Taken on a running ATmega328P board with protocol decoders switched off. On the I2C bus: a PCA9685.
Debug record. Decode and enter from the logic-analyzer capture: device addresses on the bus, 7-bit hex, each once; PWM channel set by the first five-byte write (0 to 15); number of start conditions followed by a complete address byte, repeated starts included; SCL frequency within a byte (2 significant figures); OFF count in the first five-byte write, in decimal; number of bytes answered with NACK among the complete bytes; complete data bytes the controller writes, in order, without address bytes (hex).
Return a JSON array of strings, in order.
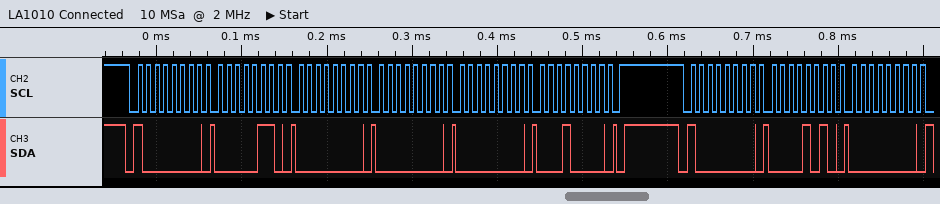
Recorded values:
["0x40", "0", "2", "100 kHz", "4096", "0", "06 00 00 00 10 0A 00"]
